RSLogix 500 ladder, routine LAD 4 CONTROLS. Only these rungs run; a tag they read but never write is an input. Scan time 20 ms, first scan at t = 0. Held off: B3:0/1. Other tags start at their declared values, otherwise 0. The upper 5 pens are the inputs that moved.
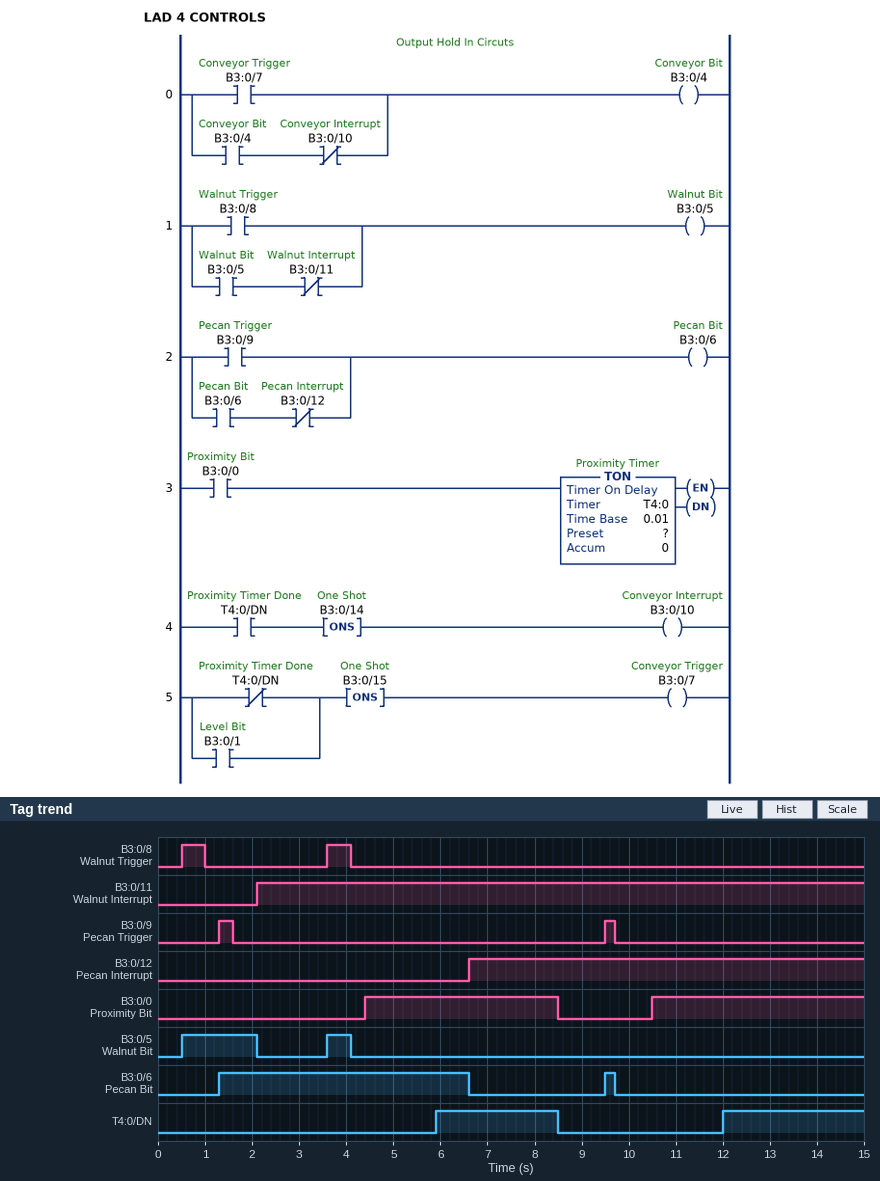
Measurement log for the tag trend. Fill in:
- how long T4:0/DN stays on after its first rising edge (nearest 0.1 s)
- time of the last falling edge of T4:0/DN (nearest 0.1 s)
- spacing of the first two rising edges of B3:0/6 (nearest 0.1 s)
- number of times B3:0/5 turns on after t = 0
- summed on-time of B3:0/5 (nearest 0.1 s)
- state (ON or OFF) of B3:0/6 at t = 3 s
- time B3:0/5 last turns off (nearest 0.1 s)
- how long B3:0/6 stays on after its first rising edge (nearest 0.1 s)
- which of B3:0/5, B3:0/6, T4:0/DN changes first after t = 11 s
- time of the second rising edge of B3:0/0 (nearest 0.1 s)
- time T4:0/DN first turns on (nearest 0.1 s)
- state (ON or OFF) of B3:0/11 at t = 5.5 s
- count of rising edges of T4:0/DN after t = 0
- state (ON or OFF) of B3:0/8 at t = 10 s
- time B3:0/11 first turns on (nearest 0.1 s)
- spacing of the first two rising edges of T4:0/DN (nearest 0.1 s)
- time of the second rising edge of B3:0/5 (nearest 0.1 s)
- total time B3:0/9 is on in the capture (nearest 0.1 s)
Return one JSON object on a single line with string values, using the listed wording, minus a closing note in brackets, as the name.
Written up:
{"how long T4:0/DN stays on after its first rising edge": "2.6 s", "time of the last falling edge of T4:0/DN": "8.5 s", "spacing of the first two rising edges of B3:0/6": "8.2 s", "number of times B3:0/5 turns on after t = 0": "2", "summed on-time of B3:0/5": "2.1 s", "state (ON or OFF) of B3:0/6 at t = 3 s": "ON", "time B3:0/5 last turns off": "4.1 s", "how long B3:0/6 stays on after its first rising edge": "5.3 s", "which of B3:0/5, B3:0/6, T4:0/DN changes first after t = 11 s": "T4:0/DN", "time of the second rising edge of B3:0/0": "10.5 s", "time T4:0/DN first turns on": "5.9 s", "state (ON or OFF) of B3:0/11 at t = 5.5 s": "ON", "count of rising edges of T4:0/DN after t = 0": "2", "state (ON or OFF) of B3:0/8 at t = 10 s": "OFF", "time B3:0/11 first turns on": "2.1 s", "spacing of the first two rising edges of T4:0/DN": "6.1 s", "time of the second rising edge of B3:0/5": "3.6 s", "total time B3:0/9 is on in the capture": "0.5 s"}
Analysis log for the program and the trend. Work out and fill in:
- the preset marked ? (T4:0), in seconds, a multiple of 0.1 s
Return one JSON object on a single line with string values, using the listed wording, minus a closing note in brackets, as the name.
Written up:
{"the preset marked ? (T4:0), in seconds, a multiple of 0.1 s": "1.5 s"}
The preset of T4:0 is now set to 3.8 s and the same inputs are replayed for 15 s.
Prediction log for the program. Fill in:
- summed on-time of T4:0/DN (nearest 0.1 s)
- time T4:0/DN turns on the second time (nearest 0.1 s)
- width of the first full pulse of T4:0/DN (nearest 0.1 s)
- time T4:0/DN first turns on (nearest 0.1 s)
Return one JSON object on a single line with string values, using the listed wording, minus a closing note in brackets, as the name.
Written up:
{"summed on-time of T4:0/DN": "1.0 s", "time T4:0/DN turns on the second time": "14.3 s", "width of the first full pulse of T4:0/DN": "0.3 s", "time T4:0/DN first turns on": "8.2 s"}
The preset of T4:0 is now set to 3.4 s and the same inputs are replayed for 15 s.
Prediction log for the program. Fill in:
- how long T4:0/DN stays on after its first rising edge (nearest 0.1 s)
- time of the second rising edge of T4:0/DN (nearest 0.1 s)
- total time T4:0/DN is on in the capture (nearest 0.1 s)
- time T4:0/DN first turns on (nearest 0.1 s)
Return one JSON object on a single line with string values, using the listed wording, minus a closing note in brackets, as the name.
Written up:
{"how long T4:0/DN stays on after its first rising edge": "0.7 s", "time of the second rising edge of T4:0/DN": "13.9 s", "total time T4:0/DN is on in the capture": "1.8 s", "time T4:0/DN first turns on": "7.8 s"}
